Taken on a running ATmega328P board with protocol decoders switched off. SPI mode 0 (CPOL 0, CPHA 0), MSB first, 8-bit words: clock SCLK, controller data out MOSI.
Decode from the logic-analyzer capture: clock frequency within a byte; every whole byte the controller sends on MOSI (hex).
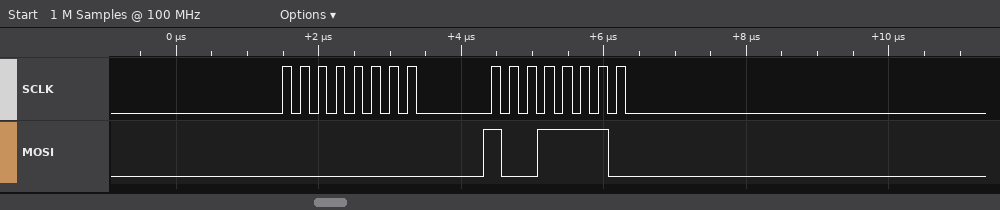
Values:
4 MHz
00 9E
